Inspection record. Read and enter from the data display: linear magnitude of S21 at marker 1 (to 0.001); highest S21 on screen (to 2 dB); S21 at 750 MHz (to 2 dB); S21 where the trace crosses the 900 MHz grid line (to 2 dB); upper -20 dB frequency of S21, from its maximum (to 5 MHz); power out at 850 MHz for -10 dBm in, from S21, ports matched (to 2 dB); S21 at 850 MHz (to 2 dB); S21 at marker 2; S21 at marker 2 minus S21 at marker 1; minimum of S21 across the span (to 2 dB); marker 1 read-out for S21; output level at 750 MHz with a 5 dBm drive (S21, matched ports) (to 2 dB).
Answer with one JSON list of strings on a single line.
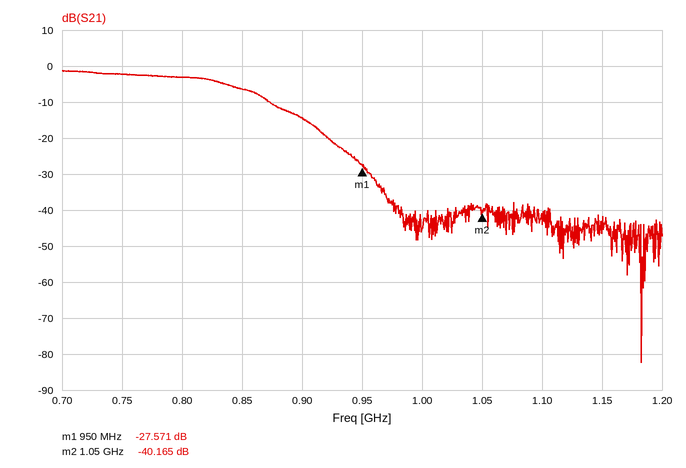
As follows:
["0.042", "-2 dB", "-2 dB", "-14 dB", "925 MHz", "-16 dBm", "-6 dB", "-40.165 dB", "-12.594 dB", "-82 dB", "-27.571 dB", "2 dBm"]
